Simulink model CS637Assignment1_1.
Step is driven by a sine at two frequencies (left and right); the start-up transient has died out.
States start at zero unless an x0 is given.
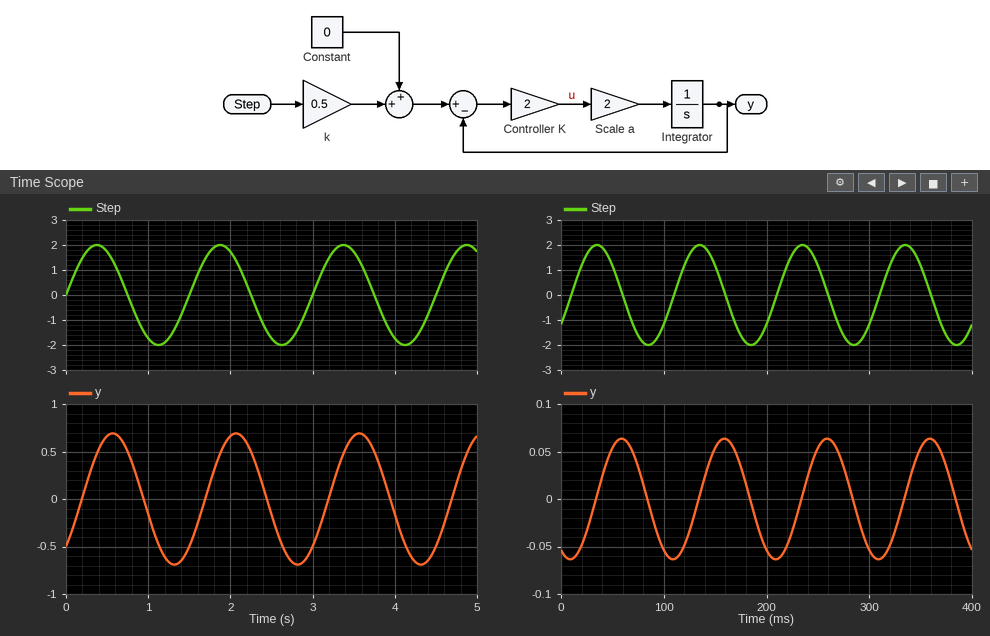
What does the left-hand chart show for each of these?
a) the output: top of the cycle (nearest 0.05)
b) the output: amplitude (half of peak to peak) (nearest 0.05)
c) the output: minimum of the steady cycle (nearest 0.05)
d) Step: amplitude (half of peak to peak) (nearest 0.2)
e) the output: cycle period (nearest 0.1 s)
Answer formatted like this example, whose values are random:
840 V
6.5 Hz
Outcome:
0.70
0.70
-0.70
2.0
1.5 s
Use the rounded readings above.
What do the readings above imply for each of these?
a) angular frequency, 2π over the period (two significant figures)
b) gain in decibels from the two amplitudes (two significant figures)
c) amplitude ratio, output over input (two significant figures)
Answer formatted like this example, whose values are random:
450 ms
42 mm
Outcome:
4.2 rad/s
-9.1 dB
0.35
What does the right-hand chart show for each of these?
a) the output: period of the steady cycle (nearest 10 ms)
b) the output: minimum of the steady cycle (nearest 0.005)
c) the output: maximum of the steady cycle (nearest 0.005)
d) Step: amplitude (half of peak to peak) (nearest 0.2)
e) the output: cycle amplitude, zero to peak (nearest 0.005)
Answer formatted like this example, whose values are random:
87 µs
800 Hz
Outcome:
100 ms
-0.065
0.065
2.0
0.065
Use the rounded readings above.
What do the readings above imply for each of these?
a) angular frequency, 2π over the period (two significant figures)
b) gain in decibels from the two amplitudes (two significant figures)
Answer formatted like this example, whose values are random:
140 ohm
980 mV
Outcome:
0.063 rad/ms
-30 dB
